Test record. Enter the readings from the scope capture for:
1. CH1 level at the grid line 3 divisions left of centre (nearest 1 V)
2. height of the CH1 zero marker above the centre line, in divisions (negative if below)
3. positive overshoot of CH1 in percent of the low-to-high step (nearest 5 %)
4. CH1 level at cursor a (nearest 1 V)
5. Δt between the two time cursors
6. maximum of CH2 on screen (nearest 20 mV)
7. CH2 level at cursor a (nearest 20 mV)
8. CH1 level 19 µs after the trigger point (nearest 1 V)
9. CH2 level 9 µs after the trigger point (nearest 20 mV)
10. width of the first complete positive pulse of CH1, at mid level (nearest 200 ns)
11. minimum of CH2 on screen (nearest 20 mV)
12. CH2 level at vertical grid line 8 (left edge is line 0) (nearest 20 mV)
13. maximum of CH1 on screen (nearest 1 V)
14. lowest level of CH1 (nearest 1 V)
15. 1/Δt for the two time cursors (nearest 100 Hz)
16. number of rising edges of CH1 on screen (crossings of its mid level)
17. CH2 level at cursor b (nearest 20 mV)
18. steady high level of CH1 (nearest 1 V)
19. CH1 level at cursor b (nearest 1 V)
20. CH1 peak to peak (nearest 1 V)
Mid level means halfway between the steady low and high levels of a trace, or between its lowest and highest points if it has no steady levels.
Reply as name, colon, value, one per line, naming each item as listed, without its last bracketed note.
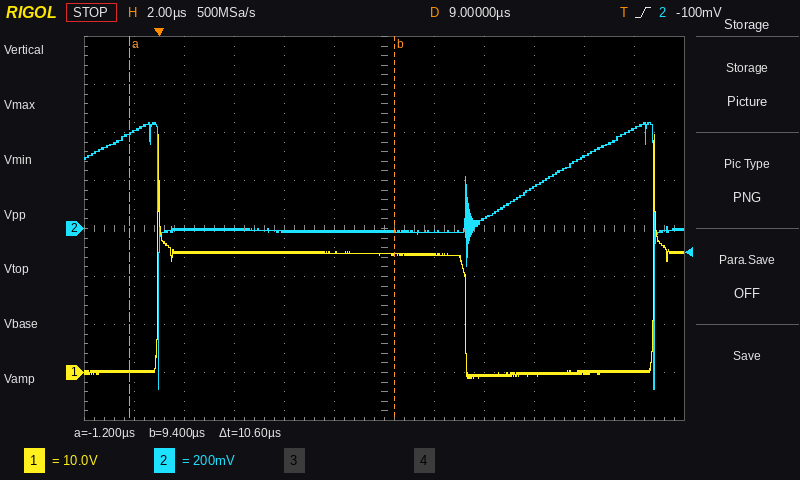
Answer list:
CH1 level at the grid line 3 divisions left of centre: 25 V
height of the CH1 zero marker above the centre line, in divisions: -3.0 div
positive overshoot of CH1 in percent of the low-to-high step: 100 %
CH1 level at cursor a: 0 V
Δt between the two time cursors: 10.6 µs
maximum of CH2 on screen: 440 mV
CH2 level at cursor a: 400 mV
CH1 level 19 µs after the trigger point: 0 V
CH2 level 9 µs after the trigger point: -20 mV
width of the first complete positive pulse of CH1, at mid level: 12.4 µs
minimum of CH2 on screen: -680 mV
CH2 level at vertical grid line 8 (left edge is line 0): 40 mV
maximum of CH1 on screen: 50 V
lowest level of CH1: -1 V
1/Δt for the two time cursors: 94.3 kHz
number of rising edges of CH1 on screen: 2
CH2 level at cursor b: -20 mV
steady high level of CH1: 25 V
CH1 level at cursor b: 25 V
CH1 peak to peak: 51 V
